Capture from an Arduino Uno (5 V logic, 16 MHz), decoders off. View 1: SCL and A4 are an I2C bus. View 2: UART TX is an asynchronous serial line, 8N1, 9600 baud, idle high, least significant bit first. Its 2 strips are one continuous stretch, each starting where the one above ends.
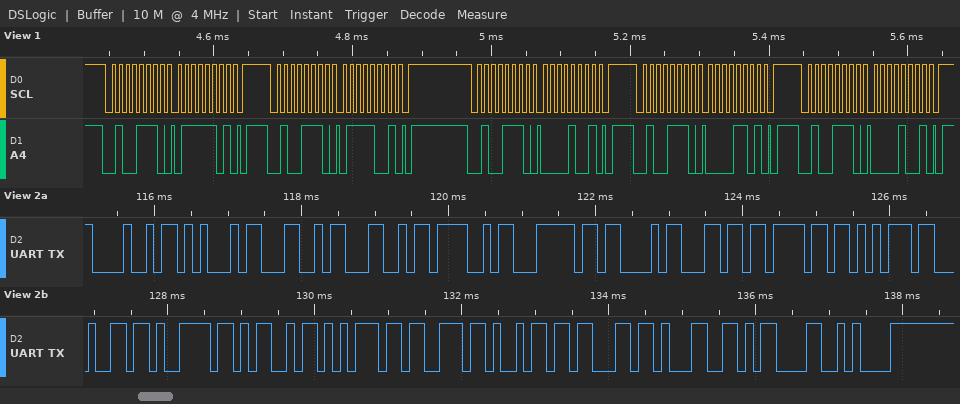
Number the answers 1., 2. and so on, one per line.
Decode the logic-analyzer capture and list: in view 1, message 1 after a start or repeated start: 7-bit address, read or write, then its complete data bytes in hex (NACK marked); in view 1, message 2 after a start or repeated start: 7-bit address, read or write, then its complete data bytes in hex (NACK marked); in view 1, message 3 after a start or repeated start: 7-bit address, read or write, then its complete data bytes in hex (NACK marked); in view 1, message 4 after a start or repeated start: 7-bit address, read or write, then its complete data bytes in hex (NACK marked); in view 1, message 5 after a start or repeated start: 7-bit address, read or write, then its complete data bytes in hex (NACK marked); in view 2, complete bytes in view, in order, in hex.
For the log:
1. 0x27 write: 7D
2. 0x27 write: 79
3. 0x27 write: 09
4. 0x27 write: 0D
5. 0x27 write: 09
6. 48 45 4C 4C 4F 7C 43 6C 6F 75 64 79 4D 75 73 69 63 31 0D 0A
